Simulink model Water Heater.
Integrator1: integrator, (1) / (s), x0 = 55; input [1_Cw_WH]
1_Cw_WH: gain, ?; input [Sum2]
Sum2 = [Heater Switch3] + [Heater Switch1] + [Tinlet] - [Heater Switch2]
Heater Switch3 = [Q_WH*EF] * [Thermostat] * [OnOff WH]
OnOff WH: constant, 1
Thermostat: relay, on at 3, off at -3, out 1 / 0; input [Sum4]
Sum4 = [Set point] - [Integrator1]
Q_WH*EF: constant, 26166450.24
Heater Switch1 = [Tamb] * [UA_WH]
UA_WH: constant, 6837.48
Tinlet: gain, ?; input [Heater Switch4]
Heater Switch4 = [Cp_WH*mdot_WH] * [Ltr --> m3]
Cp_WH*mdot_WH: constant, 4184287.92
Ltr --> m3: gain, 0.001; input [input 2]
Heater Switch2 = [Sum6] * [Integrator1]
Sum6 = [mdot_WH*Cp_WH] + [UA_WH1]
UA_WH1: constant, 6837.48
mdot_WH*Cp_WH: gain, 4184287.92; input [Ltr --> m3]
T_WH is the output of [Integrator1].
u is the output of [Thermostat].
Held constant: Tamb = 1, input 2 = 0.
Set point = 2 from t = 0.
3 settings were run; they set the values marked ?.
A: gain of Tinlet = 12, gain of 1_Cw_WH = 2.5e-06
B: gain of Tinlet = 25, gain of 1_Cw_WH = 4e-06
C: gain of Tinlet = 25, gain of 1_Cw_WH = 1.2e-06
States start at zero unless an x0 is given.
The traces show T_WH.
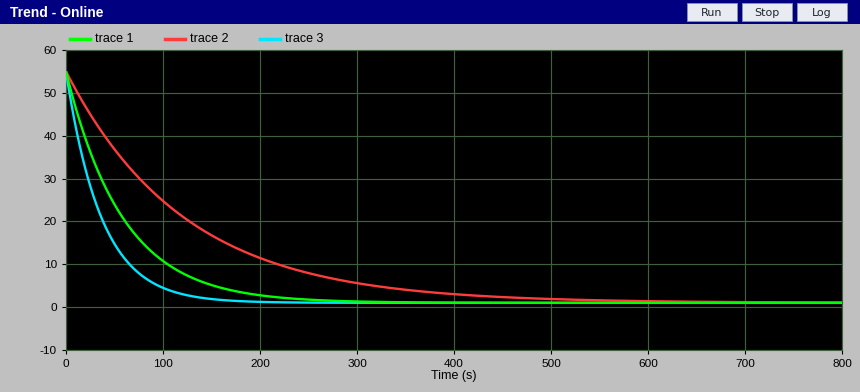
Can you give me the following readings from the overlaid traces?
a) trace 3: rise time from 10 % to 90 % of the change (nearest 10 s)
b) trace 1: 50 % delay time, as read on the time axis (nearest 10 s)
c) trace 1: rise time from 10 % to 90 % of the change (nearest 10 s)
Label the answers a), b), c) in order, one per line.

a) 80 s
b) 40 s
c) 130 s
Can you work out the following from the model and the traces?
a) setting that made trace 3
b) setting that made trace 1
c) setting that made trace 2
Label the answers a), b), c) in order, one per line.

a) B
b) A
c) C
